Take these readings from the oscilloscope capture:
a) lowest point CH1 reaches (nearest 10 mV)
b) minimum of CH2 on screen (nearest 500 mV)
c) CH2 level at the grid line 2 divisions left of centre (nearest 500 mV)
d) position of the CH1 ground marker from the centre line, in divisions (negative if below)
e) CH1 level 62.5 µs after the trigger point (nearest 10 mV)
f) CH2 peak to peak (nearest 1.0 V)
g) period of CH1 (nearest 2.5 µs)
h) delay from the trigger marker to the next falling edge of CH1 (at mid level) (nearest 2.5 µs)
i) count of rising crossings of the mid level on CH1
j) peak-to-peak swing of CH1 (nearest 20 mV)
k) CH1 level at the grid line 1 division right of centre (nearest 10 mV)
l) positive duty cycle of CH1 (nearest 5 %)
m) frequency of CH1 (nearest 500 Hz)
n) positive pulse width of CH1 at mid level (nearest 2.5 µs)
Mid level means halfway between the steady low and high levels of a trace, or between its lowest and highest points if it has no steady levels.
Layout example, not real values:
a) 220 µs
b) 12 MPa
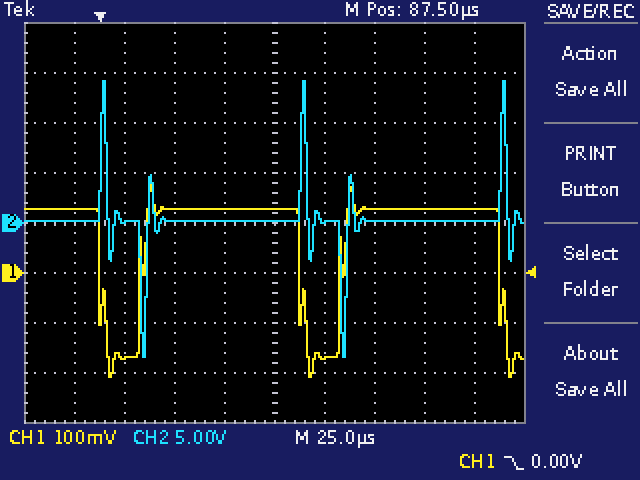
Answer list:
a) -210 mV
b) -13.5 V
c) 0.0 V
d) -1.0 div
e) 130 mV
f) 28.0 V
g) 100.0 µs
h) 100.0 µs
i) 2
j) 380 mV
k) -170 mV
l) 80 %
m) 10.0 kHz
n) 80.0 µs
